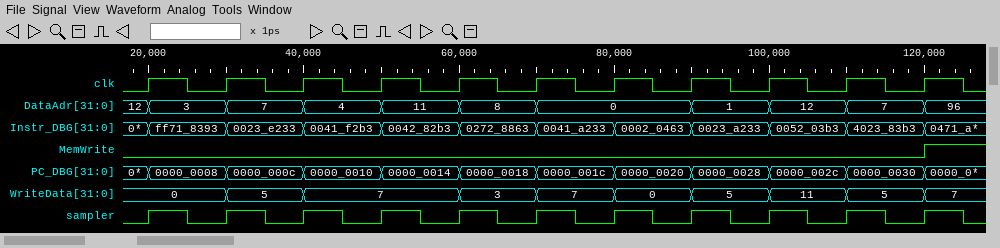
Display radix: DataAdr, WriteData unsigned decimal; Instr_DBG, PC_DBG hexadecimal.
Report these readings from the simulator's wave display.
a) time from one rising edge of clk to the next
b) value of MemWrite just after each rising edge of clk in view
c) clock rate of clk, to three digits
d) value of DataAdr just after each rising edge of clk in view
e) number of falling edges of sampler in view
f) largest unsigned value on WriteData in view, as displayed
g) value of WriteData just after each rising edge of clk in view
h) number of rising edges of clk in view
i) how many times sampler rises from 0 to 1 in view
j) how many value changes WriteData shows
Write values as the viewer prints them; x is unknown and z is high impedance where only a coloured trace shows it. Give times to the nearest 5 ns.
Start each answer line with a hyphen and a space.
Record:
- 10 ns
- 0 0 0 0 0 0 0 0 0 0 1
- 100 MHz
- 3, 7, 4, 11, 8, 0, 0, 1, 12, 7, 96
- 11
- 11
- 0, 5, 7, 7, 3, 7, 0, 5, 11, 5, 7
- 11
- 11
- 9
